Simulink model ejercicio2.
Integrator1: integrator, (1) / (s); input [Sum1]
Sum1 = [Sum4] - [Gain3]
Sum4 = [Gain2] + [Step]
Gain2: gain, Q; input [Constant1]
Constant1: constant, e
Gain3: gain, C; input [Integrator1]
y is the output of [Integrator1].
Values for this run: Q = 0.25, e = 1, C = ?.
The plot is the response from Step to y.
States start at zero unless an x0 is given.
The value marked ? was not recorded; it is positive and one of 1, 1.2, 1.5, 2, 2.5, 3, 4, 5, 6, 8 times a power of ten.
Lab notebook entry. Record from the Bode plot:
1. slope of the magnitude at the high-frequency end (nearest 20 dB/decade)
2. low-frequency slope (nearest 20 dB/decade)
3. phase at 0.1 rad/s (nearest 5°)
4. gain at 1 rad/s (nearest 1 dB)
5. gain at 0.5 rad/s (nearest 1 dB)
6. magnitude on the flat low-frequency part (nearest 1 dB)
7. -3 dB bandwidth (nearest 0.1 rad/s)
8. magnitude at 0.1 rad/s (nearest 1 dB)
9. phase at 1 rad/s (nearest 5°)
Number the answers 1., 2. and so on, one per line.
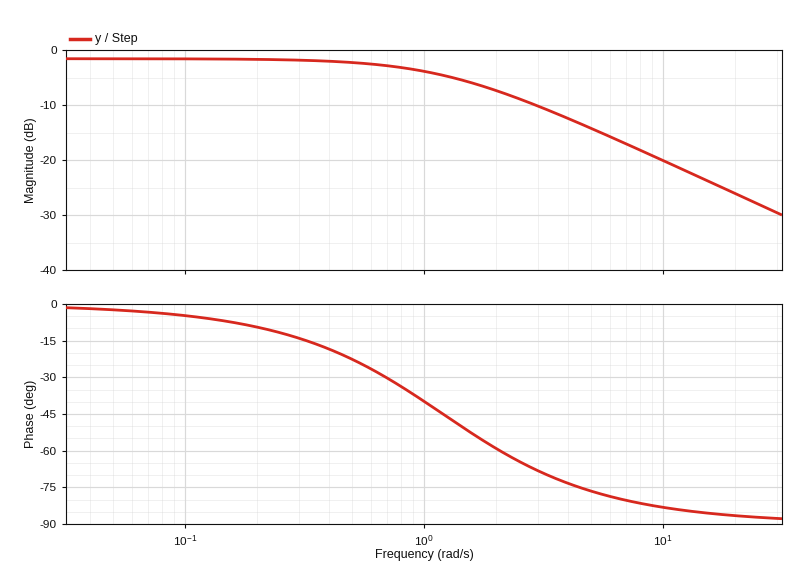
1. -20 dB/decade
2. 0 dB/decade
3. -5°
4. -4 dB
5. -2 dB
6. -2 dB
7. 1.2 rad/s
8. -2 dB
9. -40°
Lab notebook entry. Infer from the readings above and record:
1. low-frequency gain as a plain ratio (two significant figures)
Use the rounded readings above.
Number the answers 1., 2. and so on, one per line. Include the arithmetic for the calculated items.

1. 10^(-2 / 20) = 0.79
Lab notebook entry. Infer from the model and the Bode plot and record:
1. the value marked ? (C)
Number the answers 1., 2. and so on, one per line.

1. 1.2
